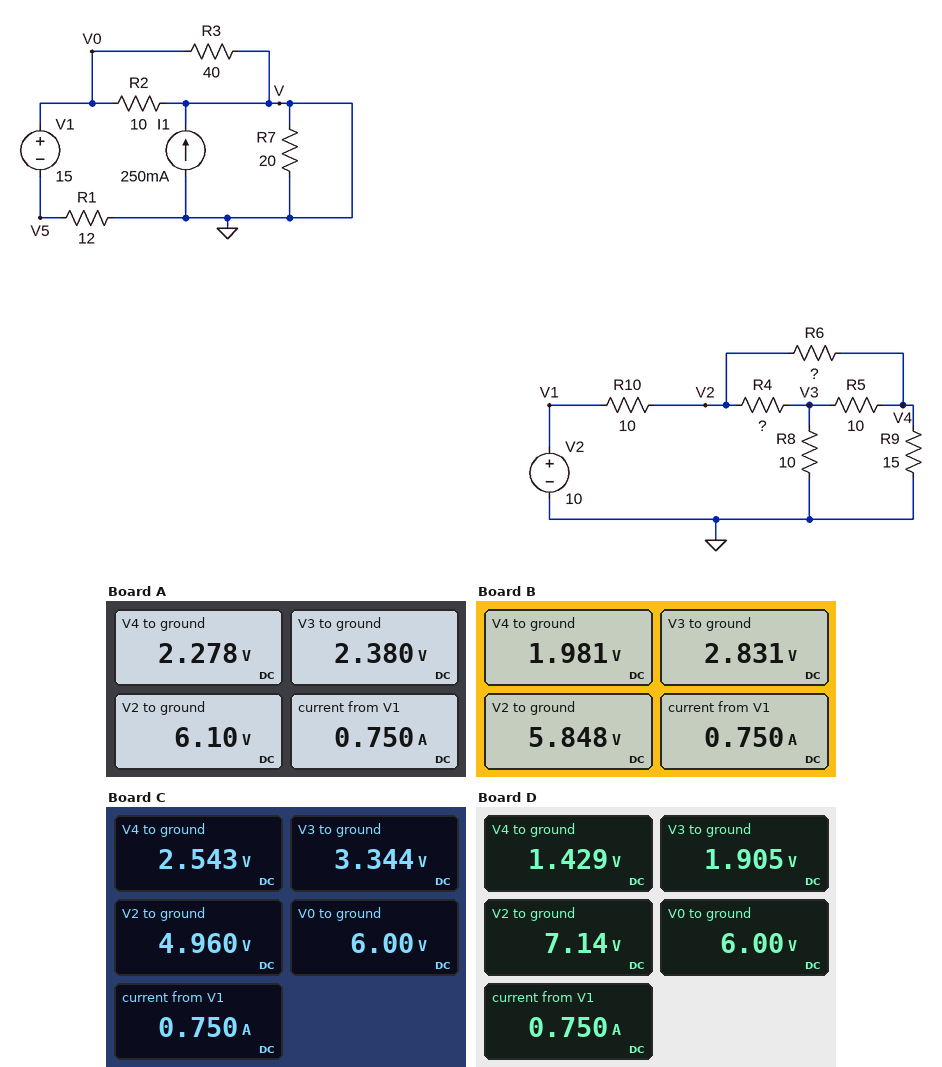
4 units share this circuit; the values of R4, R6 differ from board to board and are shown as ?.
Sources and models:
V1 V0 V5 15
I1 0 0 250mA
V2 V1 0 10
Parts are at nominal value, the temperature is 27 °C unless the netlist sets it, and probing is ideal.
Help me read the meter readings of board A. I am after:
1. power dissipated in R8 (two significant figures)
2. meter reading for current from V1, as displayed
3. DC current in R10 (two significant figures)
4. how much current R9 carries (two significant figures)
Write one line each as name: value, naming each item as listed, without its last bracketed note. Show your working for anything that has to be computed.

power dissipated in R8: (2.38 V)^2 / 10 Ω = 570 mW
meter reading for current from V1, as displayed: 0.750 A
DC current in R10: (10 V - 6.1 V) / 10 Ω = 390 mA
how much current R9 carries: (2.278 V) / 15 Ω = 150 mA
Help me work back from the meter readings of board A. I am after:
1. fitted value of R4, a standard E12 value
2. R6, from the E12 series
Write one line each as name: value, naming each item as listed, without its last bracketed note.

fitted value of R4, a standard E12 value: 15 Ω
R6, from the E12 series: 27 Ω
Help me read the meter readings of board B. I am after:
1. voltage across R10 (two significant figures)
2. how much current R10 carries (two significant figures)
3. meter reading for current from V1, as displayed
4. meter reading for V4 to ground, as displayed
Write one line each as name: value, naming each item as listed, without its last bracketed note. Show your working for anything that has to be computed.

voltage across R10: 10 V - 5.848 V = 4.2 V
how much current R10 carries: (10 V - 5.848 V) / 10 Ω = 420 mA
meter reading for current from V1, as displayed: 0.750 A
meter reading for V4 to ground, as displayed: 1.981 V
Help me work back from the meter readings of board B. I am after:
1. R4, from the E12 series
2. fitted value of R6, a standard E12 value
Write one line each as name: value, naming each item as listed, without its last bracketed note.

R4, from the E12 series: 8.2 Ω
fitted value of R6, a standard E12 value: 82 Ω
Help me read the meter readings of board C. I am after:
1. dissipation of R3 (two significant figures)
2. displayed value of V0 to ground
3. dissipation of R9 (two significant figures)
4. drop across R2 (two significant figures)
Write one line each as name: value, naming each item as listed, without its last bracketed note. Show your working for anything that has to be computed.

dissipation of R3: (6 V)^2 / 40 Ω = 900 mW
displayed value of V0 to ground: 6.00 V
dissipation of R9: (2.543 V)^2 / 15 Ω = 430 mW
drop across R2: 6 V = 6.0 V
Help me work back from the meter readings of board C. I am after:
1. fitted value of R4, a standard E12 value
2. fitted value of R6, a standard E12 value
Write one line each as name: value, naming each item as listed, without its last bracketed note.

fitted value of R4, a standard E12 value: 3.9 Ω
fitted value of R6, a standard E12 value: 27 Ω
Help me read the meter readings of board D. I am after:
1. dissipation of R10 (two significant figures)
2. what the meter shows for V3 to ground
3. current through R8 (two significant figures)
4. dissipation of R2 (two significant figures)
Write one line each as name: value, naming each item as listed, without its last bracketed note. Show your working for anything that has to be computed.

dissipation of R10: (10 V - 7.14 V)^2 / 10 Ω = 820 mW
what the meter shows for V3 to ground: 1.905 V
current through R8: (1.905 V) / 10 Ω = 190 mA
dissipation of R2: (6 V)^2 / 10 Ω = 3.6 W
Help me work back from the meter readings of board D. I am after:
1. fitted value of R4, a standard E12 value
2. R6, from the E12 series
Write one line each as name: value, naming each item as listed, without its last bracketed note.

fitted value of R4, a standard E12 value: 22 Ω
R6, from the E12 series: 120 Ω
